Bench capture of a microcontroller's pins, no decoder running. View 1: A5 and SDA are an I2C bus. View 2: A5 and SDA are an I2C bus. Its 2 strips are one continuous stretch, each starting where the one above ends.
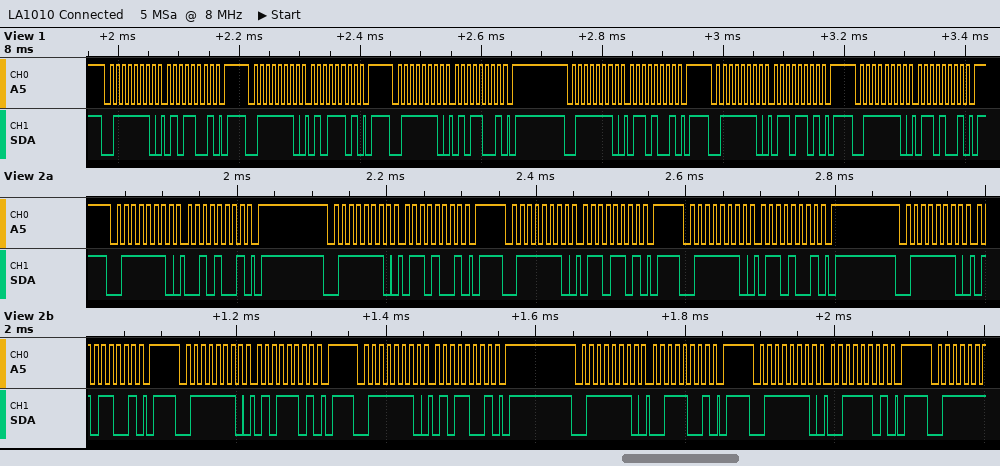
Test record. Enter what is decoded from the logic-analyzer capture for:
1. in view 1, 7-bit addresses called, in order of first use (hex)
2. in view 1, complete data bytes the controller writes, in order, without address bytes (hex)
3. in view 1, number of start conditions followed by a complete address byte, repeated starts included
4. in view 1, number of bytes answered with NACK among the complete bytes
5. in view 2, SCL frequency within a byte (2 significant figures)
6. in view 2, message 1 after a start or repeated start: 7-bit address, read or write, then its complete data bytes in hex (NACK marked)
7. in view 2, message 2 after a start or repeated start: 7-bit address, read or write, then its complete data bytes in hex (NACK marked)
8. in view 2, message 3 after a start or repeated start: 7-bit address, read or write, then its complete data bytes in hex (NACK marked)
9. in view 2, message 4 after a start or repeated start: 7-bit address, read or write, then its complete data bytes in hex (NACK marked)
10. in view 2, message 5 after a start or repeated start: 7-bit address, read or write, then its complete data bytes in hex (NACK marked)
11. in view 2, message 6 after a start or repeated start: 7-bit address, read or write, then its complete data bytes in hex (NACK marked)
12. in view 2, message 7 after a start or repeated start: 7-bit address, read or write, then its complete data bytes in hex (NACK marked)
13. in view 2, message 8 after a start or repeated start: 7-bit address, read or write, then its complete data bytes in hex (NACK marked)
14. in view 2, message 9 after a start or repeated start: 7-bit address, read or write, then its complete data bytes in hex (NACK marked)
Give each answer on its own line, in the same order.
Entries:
0x3F
59 5D 59 69 6D 69
6
0
100 kHz
0x3F write: 29
0x3F write: 69
0x3F write: 6D
0x3F write: 69
0x3F write: 59
0x3F write: 5D
0x3F write: 59
0x3F write: 39
0x3F write: 3D
